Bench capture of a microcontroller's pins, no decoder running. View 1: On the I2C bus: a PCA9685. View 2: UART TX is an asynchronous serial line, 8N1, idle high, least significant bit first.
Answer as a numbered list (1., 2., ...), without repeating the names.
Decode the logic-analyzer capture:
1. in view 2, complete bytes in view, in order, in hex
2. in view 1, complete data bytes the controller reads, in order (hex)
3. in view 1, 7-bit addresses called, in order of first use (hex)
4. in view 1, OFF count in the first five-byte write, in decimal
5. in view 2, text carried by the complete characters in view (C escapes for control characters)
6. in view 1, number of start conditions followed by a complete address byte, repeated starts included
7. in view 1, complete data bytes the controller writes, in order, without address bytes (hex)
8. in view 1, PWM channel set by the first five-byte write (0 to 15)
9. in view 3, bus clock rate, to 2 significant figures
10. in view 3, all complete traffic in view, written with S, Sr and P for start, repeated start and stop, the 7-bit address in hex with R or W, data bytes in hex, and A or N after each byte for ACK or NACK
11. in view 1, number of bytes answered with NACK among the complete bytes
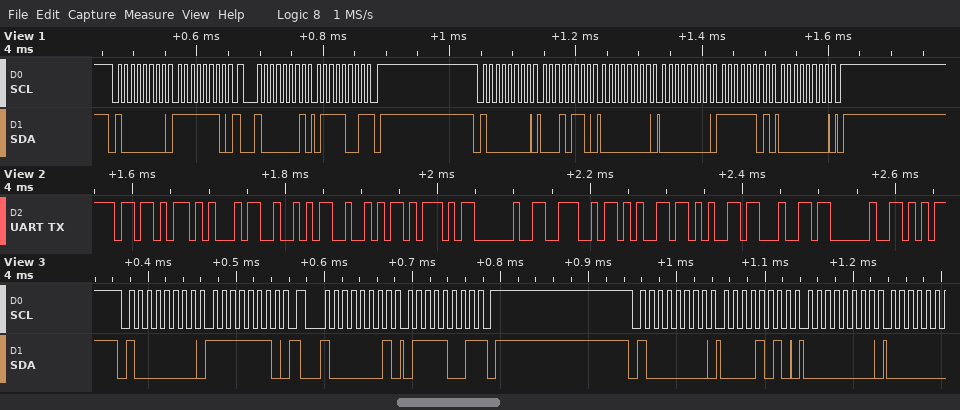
1. 5B 45 52 52 5D 20 4E 65 65 64 20
2. 79
3. 0x40
4. 253
5. "[ERR] Need "
6. 3
7. FE 16 00 00 FD 00
8. 4
9. 100 kHz
10. S 40W A FE A Sr 40R A 79 N P S 40W A 0A A 00 A
11. 1
